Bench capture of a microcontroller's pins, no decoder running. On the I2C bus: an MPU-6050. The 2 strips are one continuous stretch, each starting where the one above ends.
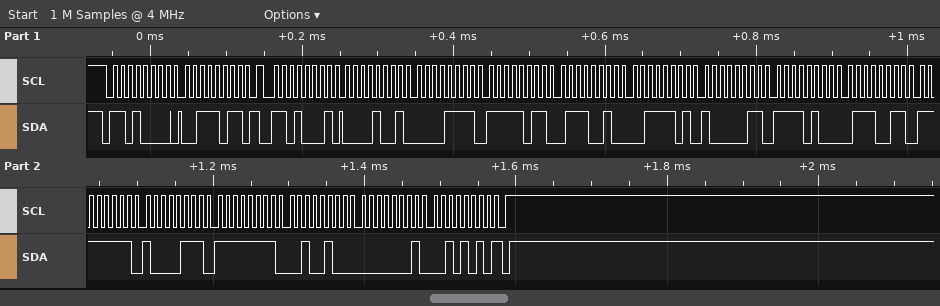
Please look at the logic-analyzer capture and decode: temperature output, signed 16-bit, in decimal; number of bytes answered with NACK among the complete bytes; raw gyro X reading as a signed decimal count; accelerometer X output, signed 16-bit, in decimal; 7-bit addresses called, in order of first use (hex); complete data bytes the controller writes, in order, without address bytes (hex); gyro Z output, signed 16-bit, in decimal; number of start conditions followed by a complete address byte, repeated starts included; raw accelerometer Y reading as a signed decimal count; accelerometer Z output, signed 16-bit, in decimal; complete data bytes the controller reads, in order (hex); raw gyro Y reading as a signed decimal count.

-2957
1
-121
2319
0x68
3B
298
2
-1166
15747
09 0F FB 72 3D 83 F4 73 FF 87 FF 24 01 2A
-220
